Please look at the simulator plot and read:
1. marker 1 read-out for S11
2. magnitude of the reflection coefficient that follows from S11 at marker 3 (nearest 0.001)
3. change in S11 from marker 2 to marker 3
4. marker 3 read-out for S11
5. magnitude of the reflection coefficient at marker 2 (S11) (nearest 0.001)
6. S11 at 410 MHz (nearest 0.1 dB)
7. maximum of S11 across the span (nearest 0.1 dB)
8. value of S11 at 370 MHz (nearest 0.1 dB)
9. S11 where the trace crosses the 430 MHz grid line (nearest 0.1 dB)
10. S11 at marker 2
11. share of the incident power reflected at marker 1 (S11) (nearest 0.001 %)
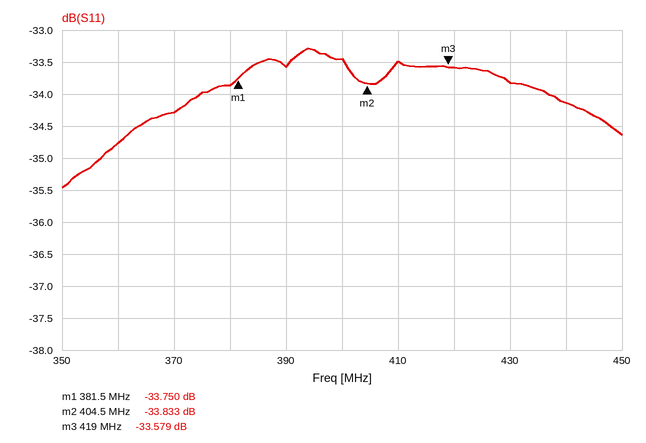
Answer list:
-33.750 dB
0.021
0.254 dB
-33.579 dB
0.020
-33.5 dB
-33.3 dB
-34.3 dB
-33.8 dB
-33.833 dB
0.042 %
